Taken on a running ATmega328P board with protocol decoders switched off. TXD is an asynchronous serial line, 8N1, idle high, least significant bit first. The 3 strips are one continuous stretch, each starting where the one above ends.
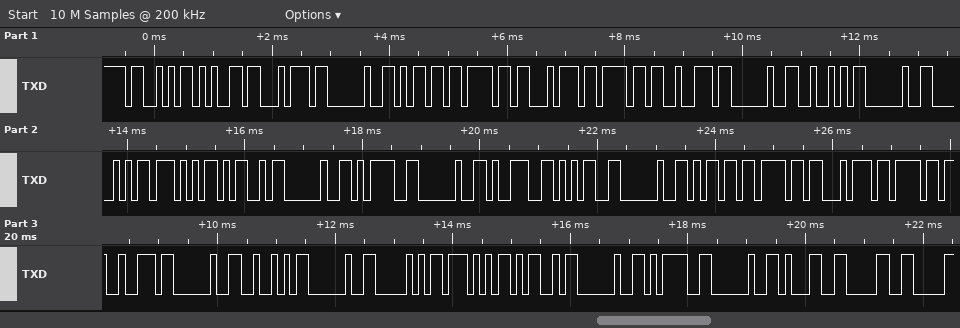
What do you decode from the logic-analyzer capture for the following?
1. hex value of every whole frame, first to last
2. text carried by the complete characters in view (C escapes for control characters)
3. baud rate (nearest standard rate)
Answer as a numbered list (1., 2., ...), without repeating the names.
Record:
1. 53 65 74 20 6D 6F 74 6F 72 20 52 20 50 57 4D 20 3D 20 39 35 20 6D 6F 74 6F 72 20 52 20 50 57 4D 20 3D 20 31 30
2. "Set motor R PWM = 95 motor R PWM = 10"
3. 9600 baud
